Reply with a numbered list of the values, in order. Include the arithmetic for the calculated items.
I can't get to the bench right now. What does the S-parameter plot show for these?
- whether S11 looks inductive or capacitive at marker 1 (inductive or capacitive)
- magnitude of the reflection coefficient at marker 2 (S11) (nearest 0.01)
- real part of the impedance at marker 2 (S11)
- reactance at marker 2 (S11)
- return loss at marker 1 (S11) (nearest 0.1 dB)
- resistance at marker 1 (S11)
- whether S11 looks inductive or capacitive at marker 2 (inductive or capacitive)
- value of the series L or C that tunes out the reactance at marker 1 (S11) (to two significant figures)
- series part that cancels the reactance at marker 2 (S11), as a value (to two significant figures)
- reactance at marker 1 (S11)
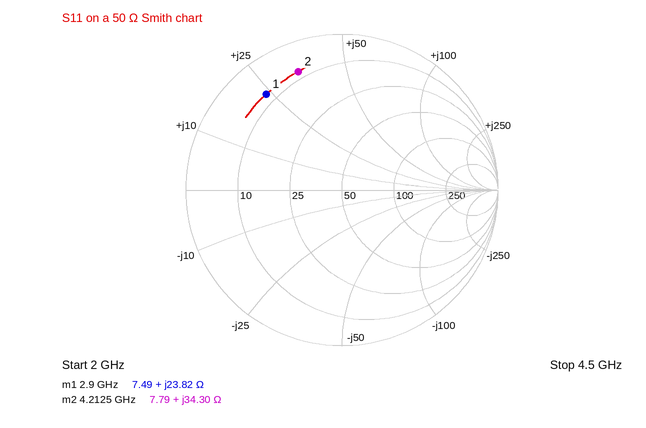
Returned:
1. inductive
2. 0.81
3. 7.79 Ω
4. +34.30 Ω
5. 2.1 dB
6. 7.49 Ω
7. inductive
8. C = 1/(2π × 2.9 GHz × 23.82 Ω) ≈ 2.3 pF
9. C = 1/(2π × 4.2125 GHz × 34.3 Ω) ≈ 1.1 pF
10. +23.82 Ω
